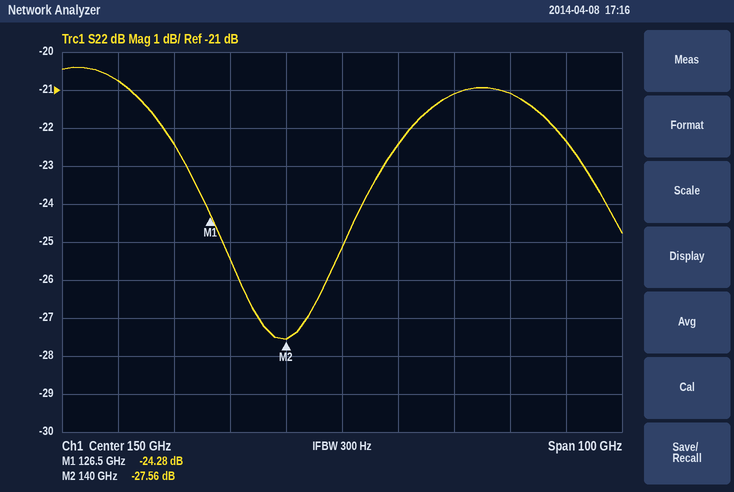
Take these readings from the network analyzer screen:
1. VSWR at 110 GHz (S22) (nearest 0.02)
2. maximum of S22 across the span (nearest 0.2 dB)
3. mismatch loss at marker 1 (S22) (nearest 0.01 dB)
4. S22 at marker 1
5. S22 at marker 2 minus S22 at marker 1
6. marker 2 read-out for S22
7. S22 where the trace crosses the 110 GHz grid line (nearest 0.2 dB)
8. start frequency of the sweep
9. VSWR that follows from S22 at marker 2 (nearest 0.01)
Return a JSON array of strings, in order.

["1.20", "-20.4 dB", "0.02 dB", "-24.28 dB", "-3.28 dB", "-27.56 dB", "-20.8 dB", "100 GHz", "1.09"]
